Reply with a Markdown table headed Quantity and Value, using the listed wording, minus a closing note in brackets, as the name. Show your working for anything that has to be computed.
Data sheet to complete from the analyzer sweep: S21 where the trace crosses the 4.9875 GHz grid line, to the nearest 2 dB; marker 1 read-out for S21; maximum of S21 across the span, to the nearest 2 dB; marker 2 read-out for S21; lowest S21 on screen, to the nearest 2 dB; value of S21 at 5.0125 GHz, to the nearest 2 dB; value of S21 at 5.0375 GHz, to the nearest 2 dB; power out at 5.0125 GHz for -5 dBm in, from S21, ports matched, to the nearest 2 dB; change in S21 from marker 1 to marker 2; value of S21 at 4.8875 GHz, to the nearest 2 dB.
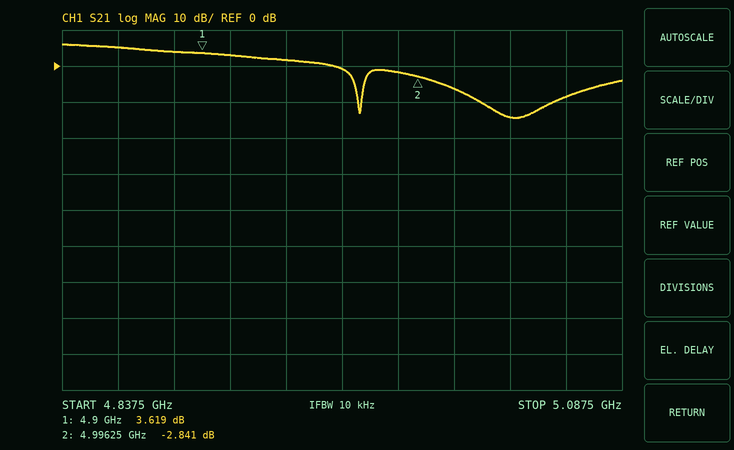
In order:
| Quantity | Value |
|---|---|
| S21 where the trace crosses the 4.9875 GHz grid line, to the nearest 2 dB | -2 dB |
| marker 1 read-out for S21 | 3.619 dB |
| maximum of S21 across the span, to the nearest 2 dB | 6 dB |
| marker 2 read-out for S21 | -2.841 dB |
| lowest S21 on screen, to the nearest 2 dB | -14 dB |
| value of S21 at 5.0125 GHz, to the nearest 2 dB | -6 dB |
| value of S21 at 5.0375 GHz, to the nearest 2 dB | -14 dB |
| power out at 5.0125 GHz for -5 dBm in, from S21, ports matched, to the nearest 2 dB | -5 dBm + (-6 dB) = -12 dBm |
| change in S21 from marker 1 to marker 2 | -2.841 − (3.619) = -6.460 dB |
| value of S21 at 4.8875 GHz, to the nearest 2 dB | 4 dB |
